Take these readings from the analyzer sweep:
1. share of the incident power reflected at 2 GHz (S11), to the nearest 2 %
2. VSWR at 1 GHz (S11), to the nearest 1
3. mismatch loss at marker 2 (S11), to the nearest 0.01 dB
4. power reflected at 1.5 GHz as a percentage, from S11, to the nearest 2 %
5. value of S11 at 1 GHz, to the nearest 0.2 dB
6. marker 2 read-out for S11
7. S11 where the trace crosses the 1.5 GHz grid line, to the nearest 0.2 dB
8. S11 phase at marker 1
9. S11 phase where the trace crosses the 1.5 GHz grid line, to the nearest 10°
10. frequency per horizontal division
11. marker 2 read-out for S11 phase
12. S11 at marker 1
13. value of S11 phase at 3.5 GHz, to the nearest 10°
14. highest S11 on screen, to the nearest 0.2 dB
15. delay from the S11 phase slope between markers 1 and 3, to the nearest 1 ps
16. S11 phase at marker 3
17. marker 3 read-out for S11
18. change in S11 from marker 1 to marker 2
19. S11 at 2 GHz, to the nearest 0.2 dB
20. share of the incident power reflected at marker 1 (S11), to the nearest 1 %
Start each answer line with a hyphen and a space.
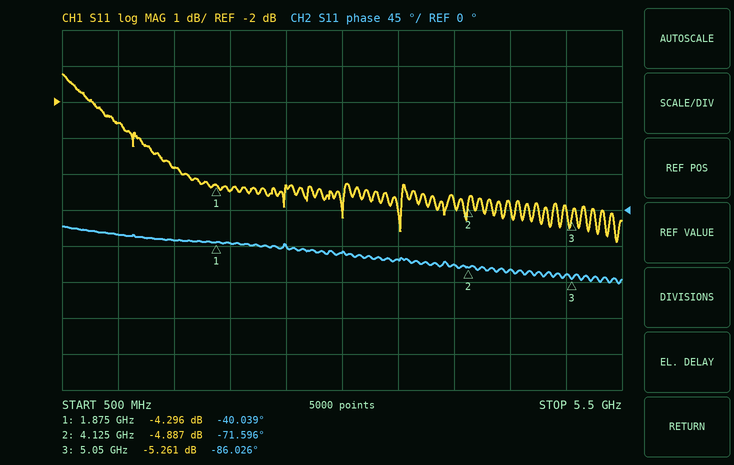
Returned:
- 36 %
- 7
- 1.70 dB
- 42 %
- -2.6 dB
- -4.887 dB
- -3.8 dB
- -40.039°
- -40°
- 500 MHz
- -71.596°
- -4.296 dB
- -60°
- -1.2 dB
- 40 ps
- -86.026°
- -5.261 dB
- -0.591 dB
- -4.4 dB
- 37 %
